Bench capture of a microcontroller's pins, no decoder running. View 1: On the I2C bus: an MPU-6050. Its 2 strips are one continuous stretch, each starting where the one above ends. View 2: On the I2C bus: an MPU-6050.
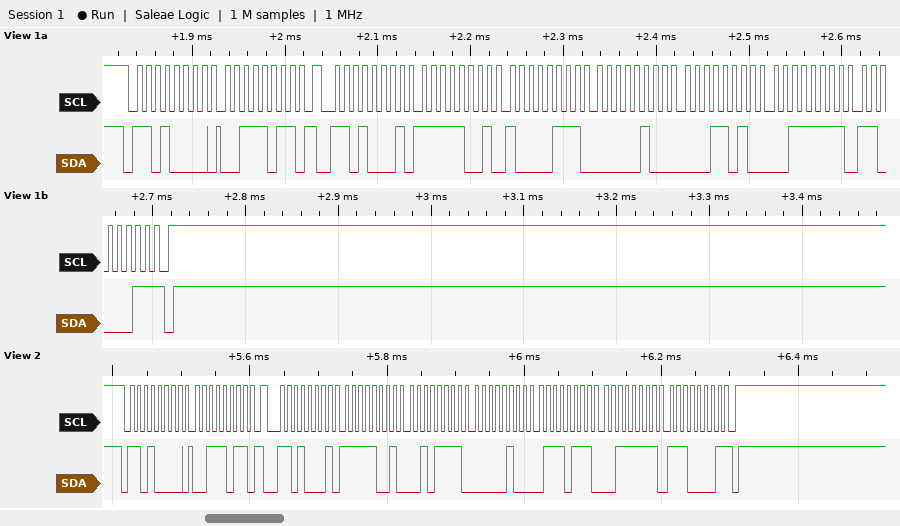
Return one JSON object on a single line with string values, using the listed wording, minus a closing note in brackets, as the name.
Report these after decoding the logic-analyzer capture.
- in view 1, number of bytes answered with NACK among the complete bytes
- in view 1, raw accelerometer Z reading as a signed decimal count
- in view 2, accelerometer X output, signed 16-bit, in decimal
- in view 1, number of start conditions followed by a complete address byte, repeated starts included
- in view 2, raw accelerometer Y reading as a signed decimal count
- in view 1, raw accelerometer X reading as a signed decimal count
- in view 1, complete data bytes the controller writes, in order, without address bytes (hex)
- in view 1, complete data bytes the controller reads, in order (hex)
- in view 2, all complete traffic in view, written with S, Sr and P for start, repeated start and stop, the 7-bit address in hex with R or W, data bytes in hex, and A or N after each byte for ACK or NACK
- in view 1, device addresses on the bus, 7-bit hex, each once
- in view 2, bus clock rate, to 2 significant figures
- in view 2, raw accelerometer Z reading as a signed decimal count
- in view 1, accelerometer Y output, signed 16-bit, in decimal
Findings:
{"in view 1, number of bytes answered with NACK among the complete bytes": "1", "in view 1, raw accelerometer Z reading as a signed decimal count": "16323", "in view 2, accelerometer X output, signed 16-bit, in decimal": "-1745", "in view 1, number of start conditions followed by a complete address byte, repeated starts included": "2", "in view 2, raw accelerometer Y reading as a signed decimal count": "1143", "in view 1, raw accelerometer X reading as a signed decimal count": "-1657", "in view 1, complete data bytes the controller writes, in order, without address bytes": "3B", "in view 1, complete data bytes the controller reads, in order": "F9 87 04 1A 3F C3", "in view 2, all complete traffic in view, written with S, Sr and P for start, repeated start and stop, the 7-bit address in hex with R or W, data bytes in hex, and A or N after each byte for ACK or NACK": "S 68W A 3B A Sr 68R A F9 A 2F A 04 A 77 A 3F A E1 N P", "in view 1, device addresses on the bus, 7-bit hex, each once": "0x68", "in view 2, bus clock rate, to 2 significant figures": "100 kHz", "in view 2, raw accelerometer Z reading as a signed decimal count": "16353", "in view 1, accelerometer Y output, signed 16-bit, in decimal": "1050"}
